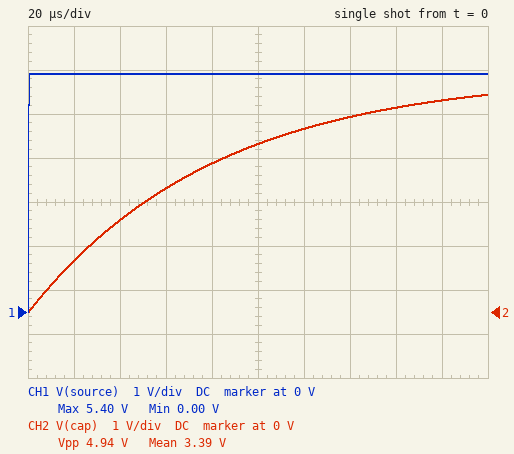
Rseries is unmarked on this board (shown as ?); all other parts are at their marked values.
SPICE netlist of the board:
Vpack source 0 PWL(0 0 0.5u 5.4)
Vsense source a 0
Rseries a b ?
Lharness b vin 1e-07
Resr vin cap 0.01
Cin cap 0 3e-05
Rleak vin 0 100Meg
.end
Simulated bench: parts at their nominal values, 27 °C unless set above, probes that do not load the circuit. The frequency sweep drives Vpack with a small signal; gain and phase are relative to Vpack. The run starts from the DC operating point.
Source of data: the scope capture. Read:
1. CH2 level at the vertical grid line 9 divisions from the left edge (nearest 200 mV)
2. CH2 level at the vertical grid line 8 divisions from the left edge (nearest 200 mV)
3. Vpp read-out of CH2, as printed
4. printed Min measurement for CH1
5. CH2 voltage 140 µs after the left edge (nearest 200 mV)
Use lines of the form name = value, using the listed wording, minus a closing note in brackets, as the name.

CH2 level at the vertical grid line 9 divisions from the left edge = 4.8 V
CH2 level at the vertical grid line 8 divisions from the left edge = 4.6 V
Vpp read-out of CH2, as printed = 4.94 V
printed Min measurement for CH1 = 0.00 V
CH2 voltage 140 µs after the left edge = 4.4 V
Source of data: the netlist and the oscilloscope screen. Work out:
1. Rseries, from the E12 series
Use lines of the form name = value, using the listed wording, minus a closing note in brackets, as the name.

Rseries, from the E12 series = 2.7 Ω
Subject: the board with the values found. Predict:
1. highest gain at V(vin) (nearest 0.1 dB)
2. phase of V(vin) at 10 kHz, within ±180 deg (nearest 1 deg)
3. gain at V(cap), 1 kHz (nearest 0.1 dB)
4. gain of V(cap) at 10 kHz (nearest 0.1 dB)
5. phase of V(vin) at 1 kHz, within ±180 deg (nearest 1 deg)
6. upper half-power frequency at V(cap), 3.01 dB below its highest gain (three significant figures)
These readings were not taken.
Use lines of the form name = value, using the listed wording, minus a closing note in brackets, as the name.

highest gain at V(vin) = 0 dB
phase of V(vin) at 10 kHz, within ±180 deg = -78 deg
gain at V(cap), 1 kHz = -1.0 dB
gain of V(cap) at 10 kHz = -14.3 dB
phase of V(vin) at 1 kHz, within ±180 deg = -27 deg
upper half-power frequency at V(cap), 3.01 dB below its highest gain = 1.96 kHz
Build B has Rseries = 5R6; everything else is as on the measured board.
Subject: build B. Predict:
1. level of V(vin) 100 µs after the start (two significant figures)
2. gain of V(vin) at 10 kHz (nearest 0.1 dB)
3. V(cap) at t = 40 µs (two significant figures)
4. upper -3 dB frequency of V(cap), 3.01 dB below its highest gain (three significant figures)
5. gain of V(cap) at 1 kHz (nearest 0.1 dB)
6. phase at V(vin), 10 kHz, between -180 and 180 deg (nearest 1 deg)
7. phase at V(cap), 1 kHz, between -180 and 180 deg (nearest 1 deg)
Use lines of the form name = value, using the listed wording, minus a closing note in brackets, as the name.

level of V(vin) 100 µs after the start = 2.4 V
gain of V(vin) at 10 kHz = -20.5 dB
V(cap) at t = 40 µs = 1.1 V
upper -3 dB frequency of V(cap), 3.01 dB below its highest gain = 946 Hz
gain of V(cap) at 1 kHz = -3.3 dB
phase at V(vin), 10 kHz, between -180 and 180 deg = -84 deg
phase at V(cap), 1 kHz, between -180 and 180 deg = -47 deg
